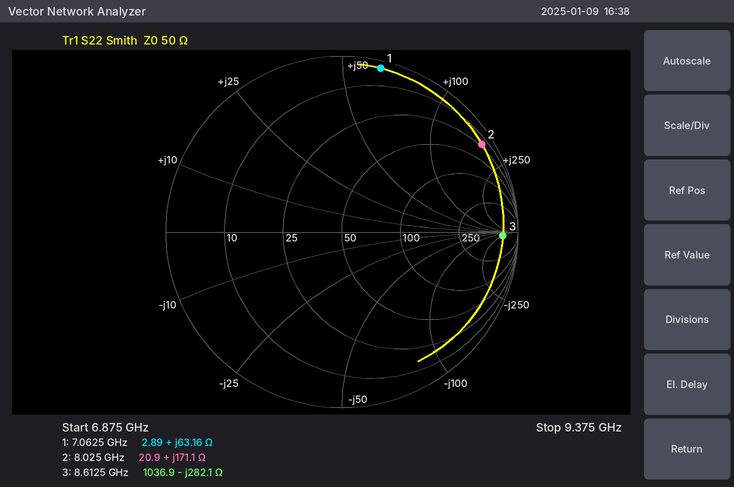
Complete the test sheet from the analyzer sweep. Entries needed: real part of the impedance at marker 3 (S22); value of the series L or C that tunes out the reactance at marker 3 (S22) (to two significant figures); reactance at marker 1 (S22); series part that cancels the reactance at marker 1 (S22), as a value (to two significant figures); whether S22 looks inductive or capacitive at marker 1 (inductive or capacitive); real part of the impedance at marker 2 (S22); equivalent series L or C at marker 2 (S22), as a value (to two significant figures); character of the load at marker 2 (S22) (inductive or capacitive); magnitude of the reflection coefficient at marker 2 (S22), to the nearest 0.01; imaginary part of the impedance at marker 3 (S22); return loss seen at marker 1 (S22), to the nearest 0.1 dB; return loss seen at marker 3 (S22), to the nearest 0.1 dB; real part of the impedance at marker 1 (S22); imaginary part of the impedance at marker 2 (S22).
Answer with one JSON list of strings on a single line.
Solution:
["1036.9 Ω", "5.2 nH", "+63.16 Ω", "360 fF", "inductive", "20.9 Ω", "3.4 nH", "inductive", "0.94", "-282.1 Ω", "0.4 dB", "0.8 dB", "2.89 Ω", "+171.1 Ω"]
